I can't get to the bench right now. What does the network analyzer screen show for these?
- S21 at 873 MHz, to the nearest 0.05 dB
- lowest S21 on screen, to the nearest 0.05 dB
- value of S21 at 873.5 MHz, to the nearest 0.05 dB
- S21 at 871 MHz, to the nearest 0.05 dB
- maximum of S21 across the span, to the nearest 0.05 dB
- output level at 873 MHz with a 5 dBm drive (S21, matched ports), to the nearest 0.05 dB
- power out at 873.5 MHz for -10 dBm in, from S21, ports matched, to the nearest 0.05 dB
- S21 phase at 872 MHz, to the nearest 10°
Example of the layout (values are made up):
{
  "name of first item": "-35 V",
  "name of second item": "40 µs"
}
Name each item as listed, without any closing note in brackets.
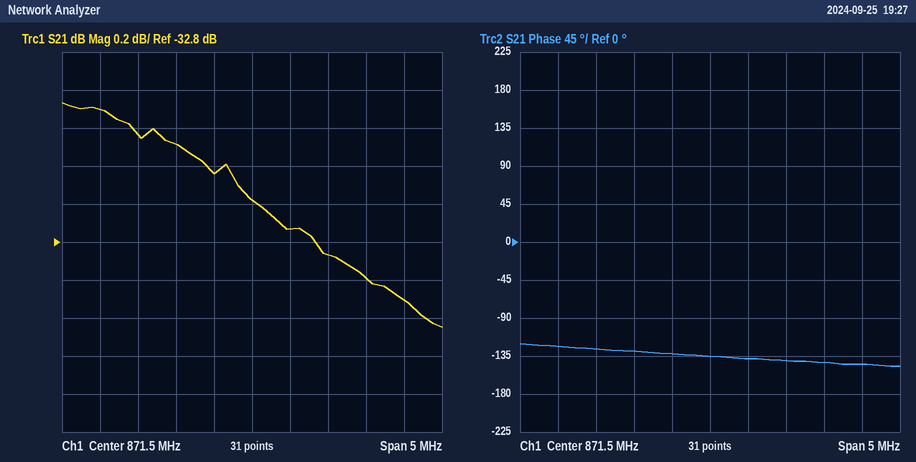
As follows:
{
  "S21 at 873 MHz, to the nearest 0.05 dB": "-33.00 dB",
  "lowest S21 on screen, to the nearest 0.05 dB": "-33.25 dB",
  "value of S21 at 873.5 MHz, to the nearest 0.05 dB": "-33.10 dB",
  "S21 at 871 MHz, to the nearest 0.05 dB": "-32.45 dB",
  "maximum of S21 across the span, to the nearest 0.05 dB": "-32.05 dB",
  "output level at 873 MHz with a 5 dBm drive (S21, matched ports), to the nearest 0.05 dB": "-28.00 dBm",
  "power out at 873.5 MHz for -10 dBm in, from S21, ports matched, to the nearest 0.05 dB": "-43.10 dBm",
  "S21 phase at 872 MHz, to the nearest 10°": "-140°"
}
